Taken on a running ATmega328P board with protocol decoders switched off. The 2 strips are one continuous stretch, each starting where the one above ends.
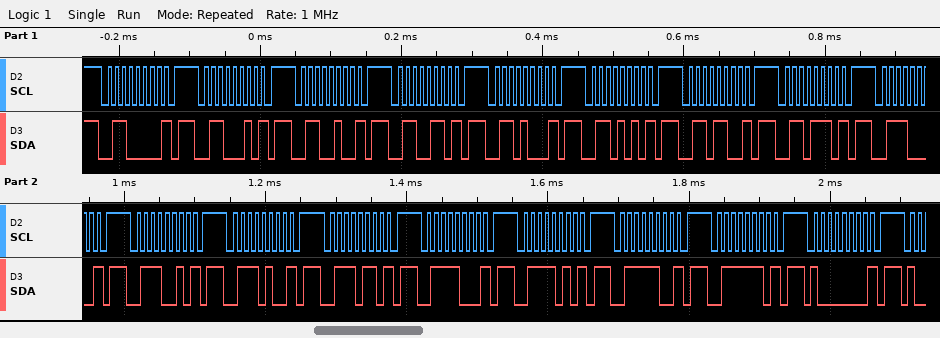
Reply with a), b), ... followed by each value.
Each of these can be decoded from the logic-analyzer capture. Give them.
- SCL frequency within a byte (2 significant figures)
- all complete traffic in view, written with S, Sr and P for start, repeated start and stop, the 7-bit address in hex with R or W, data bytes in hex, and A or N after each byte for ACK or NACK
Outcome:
a) 100 kHz
b) S 30W N P S 31W N P S 32W N P S 33W N P S 34W N P S 35W N P S 36W N P S 37W N P S 38W N P S 39W N P S 3AW N P S 3BW N P S 3CW N P S 3DW N P S 3EW N P S 3FW N P S 40W N P
